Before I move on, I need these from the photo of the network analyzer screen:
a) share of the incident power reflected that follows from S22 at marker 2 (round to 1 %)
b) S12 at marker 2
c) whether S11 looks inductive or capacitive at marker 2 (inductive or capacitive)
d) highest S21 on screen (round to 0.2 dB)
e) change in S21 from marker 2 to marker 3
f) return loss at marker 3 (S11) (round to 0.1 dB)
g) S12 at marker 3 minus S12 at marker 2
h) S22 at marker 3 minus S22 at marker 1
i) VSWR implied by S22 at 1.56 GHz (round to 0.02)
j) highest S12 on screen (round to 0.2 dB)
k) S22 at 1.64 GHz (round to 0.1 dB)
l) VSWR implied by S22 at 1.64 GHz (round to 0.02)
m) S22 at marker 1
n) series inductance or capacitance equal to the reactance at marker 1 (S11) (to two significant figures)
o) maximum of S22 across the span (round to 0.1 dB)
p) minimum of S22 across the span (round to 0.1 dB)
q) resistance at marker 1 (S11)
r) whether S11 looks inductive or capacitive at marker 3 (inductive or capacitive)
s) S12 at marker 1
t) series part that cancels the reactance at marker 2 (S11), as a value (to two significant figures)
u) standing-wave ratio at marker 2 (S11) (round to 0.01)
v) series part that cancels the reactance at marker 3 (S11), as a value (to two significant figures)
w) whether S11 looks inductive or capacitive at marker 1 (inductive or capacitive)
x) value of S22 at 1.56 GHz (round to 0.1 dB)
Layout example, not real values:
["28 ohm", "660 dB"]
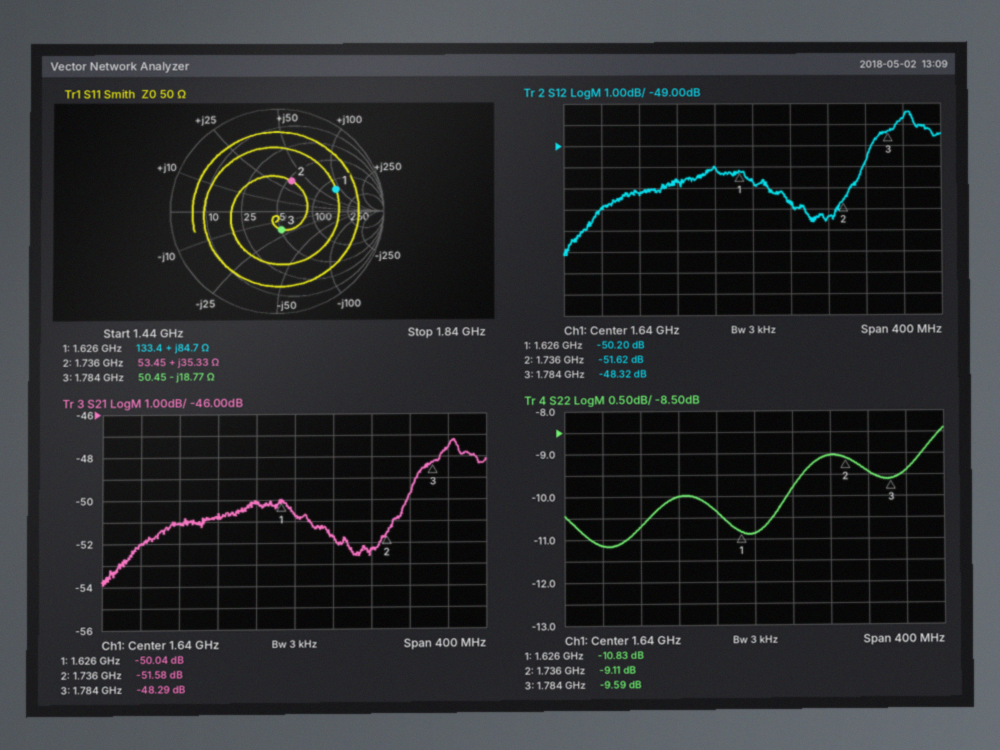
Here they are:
["12 %", "-51.62 dB", "inductive", "-47.2 dB", "3.29 dB", "14.7 dB", "3.30 dB", "1.24 dB", "1.92", "-47.4 dB", "-10.9 dB", "1.80", "-10.83 dB", "8.3 nH", "-8.4 dB", "-11.2 dB", "133.4 Ω", "capacitive", "-50.20 dB", "2.6 pF", "1.96", "1.7 nH", "inductive", "-10.0 dB"]
